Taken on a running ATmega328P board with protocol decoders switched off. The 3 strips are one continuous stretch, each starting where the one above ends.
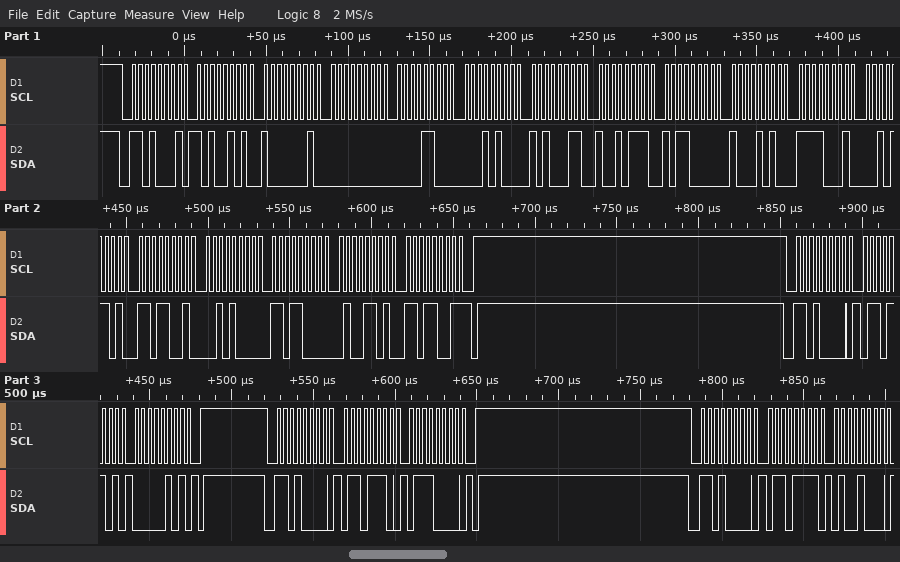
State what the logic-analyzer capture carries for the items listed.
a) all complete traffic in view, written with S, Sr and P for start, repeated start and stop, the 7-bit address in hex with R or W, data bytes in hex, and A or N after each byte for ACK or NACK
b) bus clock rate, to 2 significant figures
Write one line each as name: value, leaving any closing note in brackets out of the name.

all complete traffic in view, written with S, Sr and P for start, repeated start and stop, the 7-bit address in hex with R or W, data bytes in hex, and A or N after each byte for ACK or NACK: S 68R A A5 A 81 A 00 A 0C A 14 A A3 A 97 A B0 A 8A A F1 A 2D A D9 A 28 A D8 A 4D A D9 N P S 68W A 6D A 05 A P S 68W A 6E A 70 A P S 68W A 6F A 48 A
bus clock rate, to 2 significant figures: 250 kHz
